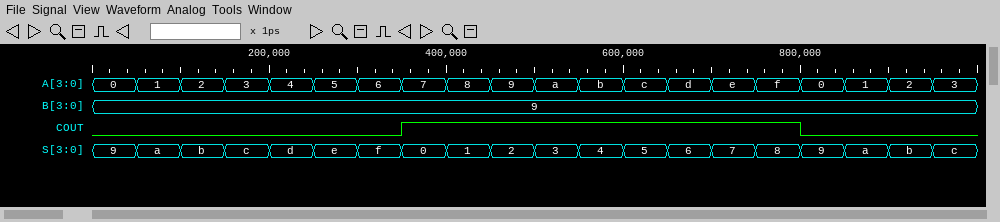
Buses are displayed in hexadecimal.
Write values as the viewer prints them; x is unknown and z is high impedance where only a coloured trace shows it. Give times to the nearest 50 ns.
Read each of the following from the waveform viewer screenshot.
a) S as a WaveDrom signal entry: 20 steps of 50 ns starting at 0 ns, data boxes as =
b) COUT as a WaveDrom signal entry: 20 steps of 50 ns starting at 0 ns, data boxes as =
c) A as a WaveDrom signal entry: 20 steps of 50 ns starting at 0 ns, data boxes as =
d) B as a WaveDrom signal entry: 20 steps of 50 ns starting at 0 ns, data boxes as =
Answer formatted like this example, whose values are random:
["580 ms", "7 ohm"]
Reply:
["{name: 'S', wave: '====================', data: '9 a b c d e f 0 1 2 3 4 5 6 7 8 9 a b c'}", "{name: 'COUT', wave: '0......1........0...'}", "{name: 'A', wave: '====================', data: '0 1 2 3 4 5 6 7 8 9 a b c d e f 0 1 2 3'}", "{name: 'B', wave: '=...................', data: '9'}"]
